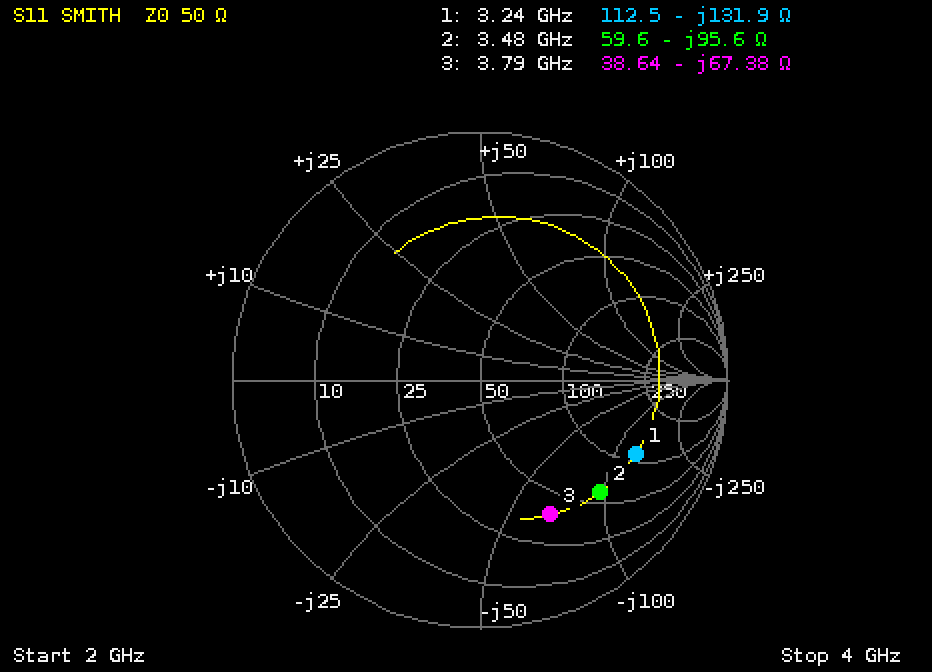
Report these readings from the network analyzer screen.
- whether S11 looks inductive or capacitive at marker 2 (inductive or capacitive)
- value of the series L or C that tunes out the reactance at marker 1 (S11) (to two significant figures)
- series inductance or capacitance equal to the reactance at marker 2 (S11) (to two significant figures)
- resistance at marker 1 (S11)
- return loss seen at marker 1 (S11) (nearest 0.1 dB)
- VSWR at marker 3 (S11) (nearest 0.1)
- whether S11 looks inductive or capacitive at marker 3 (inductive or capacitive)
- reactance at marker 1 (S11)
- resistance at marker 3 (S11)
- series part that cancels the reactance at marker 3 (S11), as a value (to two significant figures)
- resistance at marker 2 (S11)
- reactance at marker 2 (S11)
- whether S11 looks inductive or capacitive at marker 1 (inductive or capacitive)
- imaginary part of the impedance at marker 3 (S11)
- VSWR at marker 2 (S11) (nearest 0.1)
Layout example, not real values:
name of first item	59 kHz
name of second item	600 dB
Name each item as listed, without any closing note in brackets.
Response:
whether S11 looks inductive or capacitive at marker 2	capacitive
value of the series L or C that tunes out the reactance at marker 1 (S11)	6.5 nH
series inductance or capacitance equal to the reactance at marker 2 (S11)	480 fF
resistance at marker 1	112.5 Ω
return loss seen at marker 1 (S11)	3.1 dB
VSWR at marker 3 (S11)	4.2
whether S11 looks inductive or capacitive at marker 3	capacitive
reactance at marker 1	-131.9 Ω
resistance at marker 3	38.64 Ω
series part that cancels the reactance at marker 3 (S11), as a value	2.8 nH
resistance at marker 2	59.6 Ω
reactance at marker 2	-95.6 Ω
whether S11 looks inductive or capacitive at marker 1	capacitive
imaginary part of the impedance at marker 3	-67.38 Ω
VSWR at marker 2 (S11)	4.9
